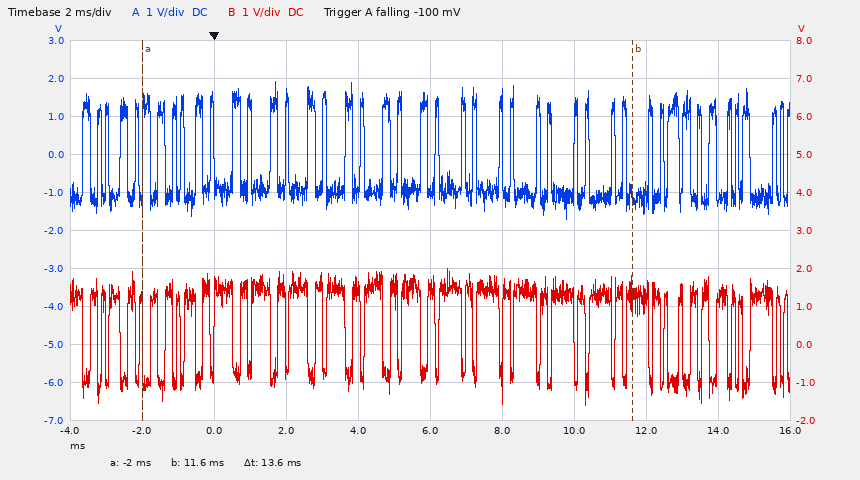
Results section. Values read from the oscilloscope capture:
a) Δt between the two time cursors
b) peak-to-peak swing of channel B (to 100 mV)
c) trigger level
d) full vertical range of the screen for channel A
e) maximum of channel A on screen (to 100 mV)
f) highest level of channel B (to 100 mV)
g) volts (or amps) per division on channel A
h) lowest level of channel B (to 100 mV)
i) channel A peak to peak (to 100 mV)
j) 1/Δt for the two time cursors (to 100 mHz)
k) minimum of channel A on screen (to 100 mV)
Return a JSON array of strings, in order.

["13.6 ms", "3.6 V", "-100 mV", "10 V", "1.9 V", "2.0 V", "1 V", "-1.6 V", "3.6 V", "73.5 Hz", "-1.7 V"]
